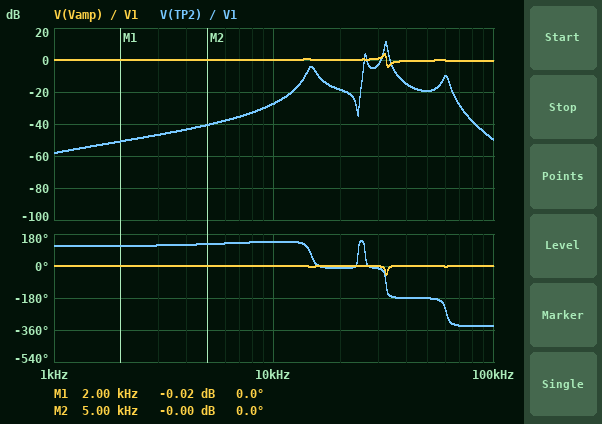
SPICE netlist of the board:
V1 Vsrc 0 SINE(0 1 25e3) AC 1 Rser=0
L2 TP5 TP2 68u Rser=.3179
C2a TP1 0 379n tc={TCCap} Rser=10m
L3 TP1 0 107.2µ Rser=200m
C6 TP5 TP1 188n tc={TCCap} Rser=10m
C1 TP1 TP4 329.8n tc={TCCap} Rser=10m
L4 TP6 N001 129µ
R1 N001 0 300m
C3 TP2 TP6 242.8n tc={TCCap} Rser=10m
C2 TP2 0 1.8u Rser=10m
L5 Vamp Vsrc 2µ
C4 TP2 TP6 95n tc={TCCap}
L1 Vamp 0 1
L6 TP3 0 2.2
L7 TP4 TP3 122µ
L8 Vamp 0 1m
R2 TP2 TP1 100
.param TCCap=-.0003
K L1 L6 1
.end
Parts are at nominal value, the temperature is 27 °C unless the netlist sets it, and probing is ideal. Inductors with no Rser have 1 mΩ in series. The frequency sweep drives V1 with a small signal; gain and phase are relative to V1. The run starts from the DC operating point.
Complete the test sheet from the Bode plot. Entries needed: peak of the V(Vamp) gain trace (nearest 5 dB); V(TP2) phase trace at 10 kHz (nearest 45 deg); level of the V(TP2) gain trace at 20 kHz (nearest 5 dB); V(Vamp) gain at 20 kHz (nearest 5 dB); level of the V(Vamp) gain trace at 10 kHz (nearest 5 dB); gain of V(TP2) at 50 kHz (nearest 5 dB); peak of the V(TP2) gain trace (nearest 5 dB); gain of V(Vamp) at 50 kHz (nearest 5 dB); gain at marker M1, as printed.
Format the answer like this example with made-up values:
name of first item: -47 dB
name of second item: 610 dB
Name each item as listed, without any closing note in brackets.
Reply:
peak of the V(Vamp) gain trace: 5 dB
V(TP2) phase trace at 10 kHz: 135 deg
level of the V(TP2) gain trace at 20 kHz: -20 dB
V(Vamp) gain at 20 kHz: 0 dB
level of the V(Vamp) gain trace at 10 kHz: 0 dB
gain of V(TP2) at 50 kHz: -20 dB
peak of the V(TP2) gain trace: 10 dB
gain of V(Vamp) at 50 kHz: 0 dB
gain at marker M1, as printed: -0.02 dB
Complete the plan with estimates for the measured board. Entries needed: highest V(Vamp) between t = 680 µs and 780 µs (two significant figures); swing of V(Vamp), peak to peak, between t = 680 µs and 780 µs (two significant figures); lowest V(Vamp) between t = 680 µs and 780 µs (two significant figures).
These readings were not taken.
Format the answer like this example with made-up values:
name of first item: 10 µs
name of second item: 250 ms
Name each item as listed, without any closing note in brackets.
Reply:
highest V(Vamp) between t = 680 µs and 780 µs: 1.0 V
swing of V(Vamp), peak to peak, between t = 680 µs and 780 µs: 2.1 V
lowest V(Vamp) between t = 680 µs and 780 µs: -1.0 V
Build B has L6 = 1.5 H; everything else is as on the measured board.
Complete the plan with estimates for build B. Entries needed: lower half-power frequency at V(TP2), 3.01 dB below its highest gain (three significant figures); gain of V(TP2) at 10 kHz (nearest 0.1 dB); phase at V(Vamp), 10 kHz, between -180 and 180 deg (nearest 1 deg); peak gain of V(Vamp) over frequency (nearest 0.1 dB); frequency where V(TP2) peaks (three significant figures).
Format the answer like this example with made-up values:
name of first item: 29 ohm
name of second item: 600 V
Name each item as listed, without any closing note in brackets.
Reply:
lower half-power frequency at V(TP2), 3.01 dB below its highest gain: 32.0 kHz
gain of V(TP2) at 10 kHz: -28.9 dB
phase at V(Vamp), 10 kHz, between -180 and 180 deg: 0 deg
peak gain of V(Vamp) over frequency: 2.7 dB
frequency where V(TP2) peaks: 32.4 kHz
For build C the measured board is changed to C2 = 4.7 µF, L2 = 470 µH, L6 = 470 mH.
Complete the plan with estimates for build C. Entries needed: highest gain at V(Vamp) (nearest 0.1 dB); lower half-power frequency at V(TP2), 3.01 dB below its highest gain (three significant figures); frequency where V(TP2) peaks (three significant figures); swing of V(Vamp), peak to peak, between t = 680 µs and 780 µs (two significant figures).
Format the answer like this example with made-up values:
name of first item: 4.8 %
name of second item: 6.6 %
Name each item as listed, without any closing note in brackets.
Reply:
highest gain at V(Vamp): 0.4 dB
lower half-power frequency at V(TP2), 3.01 dB below its highest gain: 19.3 kHz
frequency where V(TP2) peaks: 19.6 kHz
swing of V(Vamp), peak to peak, between t = 680 µs and 780 µs: 2.0 V
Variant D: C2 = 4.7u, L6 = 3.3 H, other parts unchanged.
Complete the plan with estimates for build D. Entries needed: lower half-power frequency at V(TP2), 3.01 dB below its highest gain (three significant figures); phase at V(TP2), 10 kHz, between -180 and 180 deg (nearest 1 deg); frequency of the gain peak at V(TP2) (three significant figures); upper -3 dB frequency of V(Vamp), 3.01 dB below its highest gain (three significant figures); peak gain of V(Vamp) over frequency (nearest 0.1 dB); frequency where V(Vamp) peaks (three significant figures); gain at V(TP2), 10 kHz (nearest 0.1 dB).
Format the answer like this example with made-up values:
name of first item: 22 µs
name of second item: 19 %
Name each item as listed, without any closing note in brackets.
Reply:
lower half-power frequency at V(TP2), 3.01 dB below its highest gain: 31.1 kHz
phase at V(TP2), 10 kHz, between -180 and 180 deg: 134 deg
frequency of the gain peak at V(TP2): 31.6 kHz
upper -3 dB frequency of V(Vamp), 3.01 dB below its highest gain: 31.7 kHz
peak gain of V(Vamp) over frequency: 4.5 dB
frequency where V(Vamp) peaks: 31.3 kHz
gain at V(TP2), 10 kHz: -32.2 dB
